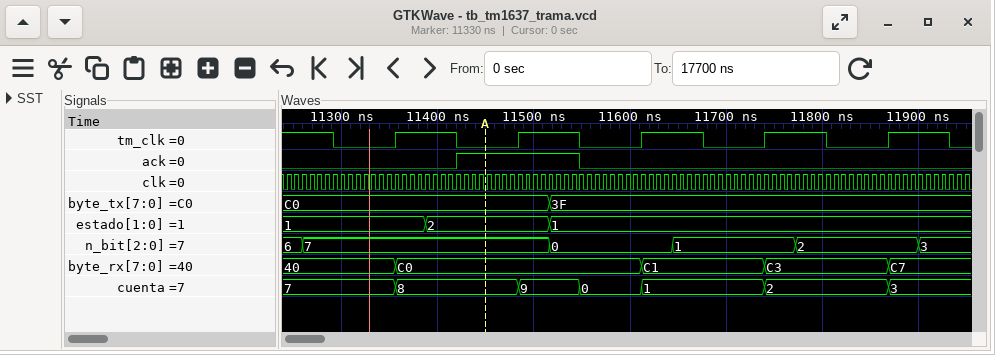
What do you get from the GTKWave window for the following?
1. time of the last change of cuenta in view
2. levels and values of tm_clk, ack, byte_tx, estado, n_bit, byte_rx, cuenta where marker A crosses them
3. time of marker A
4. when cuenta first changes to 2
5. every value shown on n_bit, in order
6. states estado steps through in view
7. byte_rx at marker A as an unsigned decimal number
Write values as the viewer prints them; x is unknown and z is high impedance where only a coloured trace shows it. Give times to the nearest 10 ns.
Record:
11870 ns
tm_clk=0, ack=1, byte_tx=C0, estado=2, n_bit=7, byte_rx=C0, cuenta=8
11450 ns
11740 ns
6, 7, 0, 1, 2, 3
1, 2, 1
192
